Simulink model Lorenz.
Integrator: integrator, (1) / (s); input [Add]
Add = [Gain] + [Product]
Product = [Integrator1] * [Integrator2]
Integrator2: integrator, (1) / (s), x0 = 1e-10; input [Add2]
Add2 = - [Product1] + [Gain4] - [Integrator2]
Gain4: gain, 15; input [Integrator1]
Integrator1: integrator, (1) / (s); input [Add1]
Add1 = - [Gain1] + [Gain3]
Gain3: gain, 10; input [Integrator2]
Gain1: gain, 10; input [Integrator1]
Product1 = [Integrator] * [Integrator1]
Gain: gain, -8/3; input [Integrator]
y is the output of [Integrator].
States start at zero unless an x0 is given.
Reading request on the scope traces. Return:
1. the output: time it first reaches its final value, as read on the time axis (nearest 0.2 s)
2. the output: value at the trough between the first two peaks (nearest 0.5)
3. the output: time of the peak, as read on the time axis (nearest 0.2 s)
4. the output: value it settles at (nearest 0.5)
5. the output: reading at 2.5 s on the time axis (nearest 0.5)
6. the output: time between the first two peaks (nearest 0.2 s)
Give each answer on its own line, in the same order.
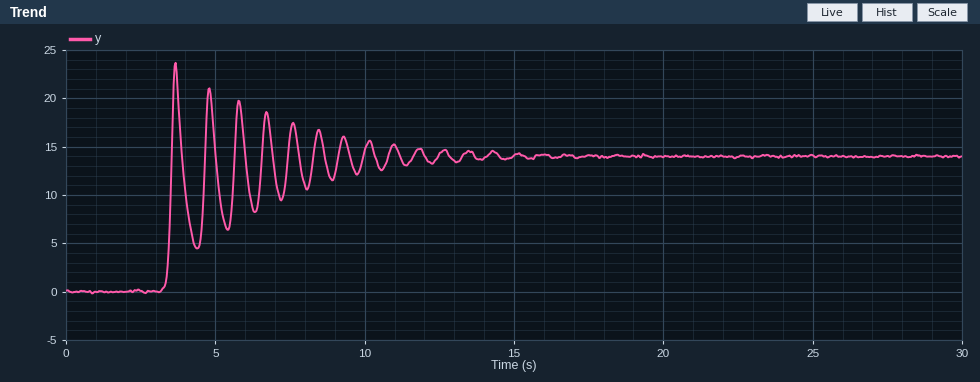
3.6 s
4.5
3.6 s
14.0
0.0
1.2 s
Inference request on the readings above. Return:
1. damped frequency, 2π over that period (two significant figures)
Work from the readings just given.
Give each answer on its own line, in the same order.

5.2 rad/s
